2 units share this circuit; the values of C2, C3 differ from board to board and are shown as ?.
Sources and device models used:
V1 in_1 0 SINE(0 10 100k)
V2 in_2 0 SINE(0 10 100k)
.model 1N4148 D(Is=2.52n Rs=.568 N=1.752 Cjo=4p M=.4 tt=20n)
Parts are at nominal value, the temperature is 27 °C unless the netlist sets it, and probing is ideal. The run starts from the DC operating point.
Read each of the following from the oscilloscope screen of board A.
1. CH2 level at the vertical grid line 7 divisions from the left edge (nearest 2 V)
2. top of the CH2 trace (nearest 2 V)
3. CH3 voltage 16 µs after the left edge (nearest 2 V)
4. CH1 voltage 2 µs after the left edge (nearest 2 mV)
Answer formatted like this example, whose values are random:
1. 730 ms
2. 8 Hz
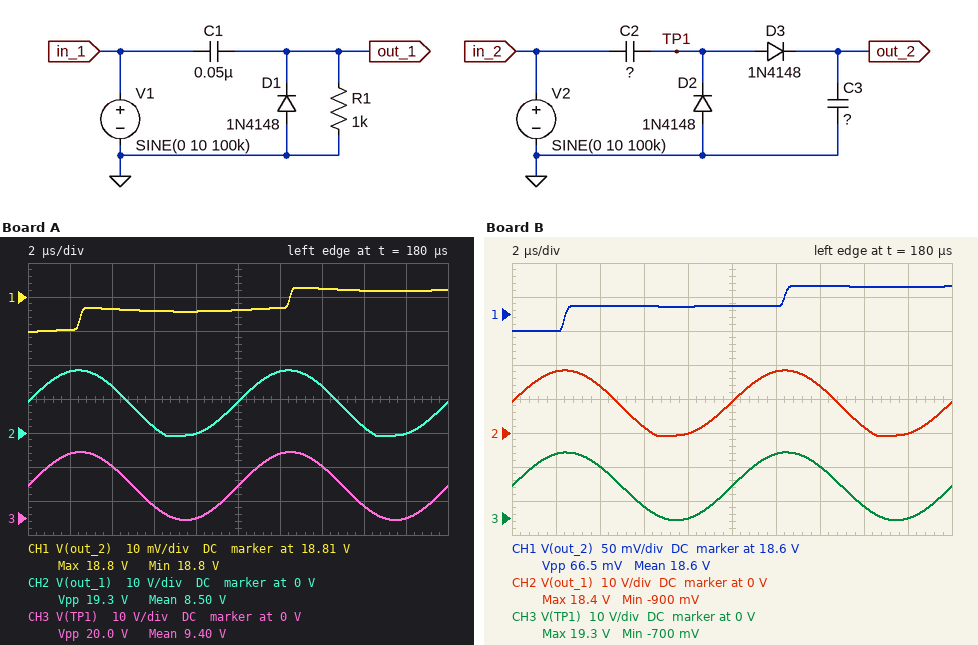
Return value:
1. 14 V
2. 18 V
3. 4 V
4. 18.800 V
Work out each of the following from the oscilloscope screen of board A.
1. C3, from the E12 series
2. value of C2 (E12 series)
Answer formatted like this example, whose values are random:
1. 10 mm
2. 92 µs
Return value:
1. 33 nF
2. 120 nF
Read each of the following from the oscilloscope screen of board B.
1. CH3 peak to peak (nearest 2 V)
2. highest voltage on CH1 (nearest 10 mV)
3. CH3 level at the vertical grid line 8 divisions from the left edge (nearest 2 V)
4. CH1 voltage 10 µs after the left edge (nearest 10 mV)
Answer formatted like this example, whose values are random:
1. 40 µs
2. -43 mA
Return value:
1. 20 V
2. 18.64 V
3. 4 V
4. 18.61 V
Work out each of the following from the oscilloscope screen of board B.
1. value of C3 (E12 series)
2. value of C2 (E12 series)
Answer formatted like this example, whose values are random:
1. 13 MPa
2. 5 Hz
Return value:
1. 56 nF
2. 18 nF
